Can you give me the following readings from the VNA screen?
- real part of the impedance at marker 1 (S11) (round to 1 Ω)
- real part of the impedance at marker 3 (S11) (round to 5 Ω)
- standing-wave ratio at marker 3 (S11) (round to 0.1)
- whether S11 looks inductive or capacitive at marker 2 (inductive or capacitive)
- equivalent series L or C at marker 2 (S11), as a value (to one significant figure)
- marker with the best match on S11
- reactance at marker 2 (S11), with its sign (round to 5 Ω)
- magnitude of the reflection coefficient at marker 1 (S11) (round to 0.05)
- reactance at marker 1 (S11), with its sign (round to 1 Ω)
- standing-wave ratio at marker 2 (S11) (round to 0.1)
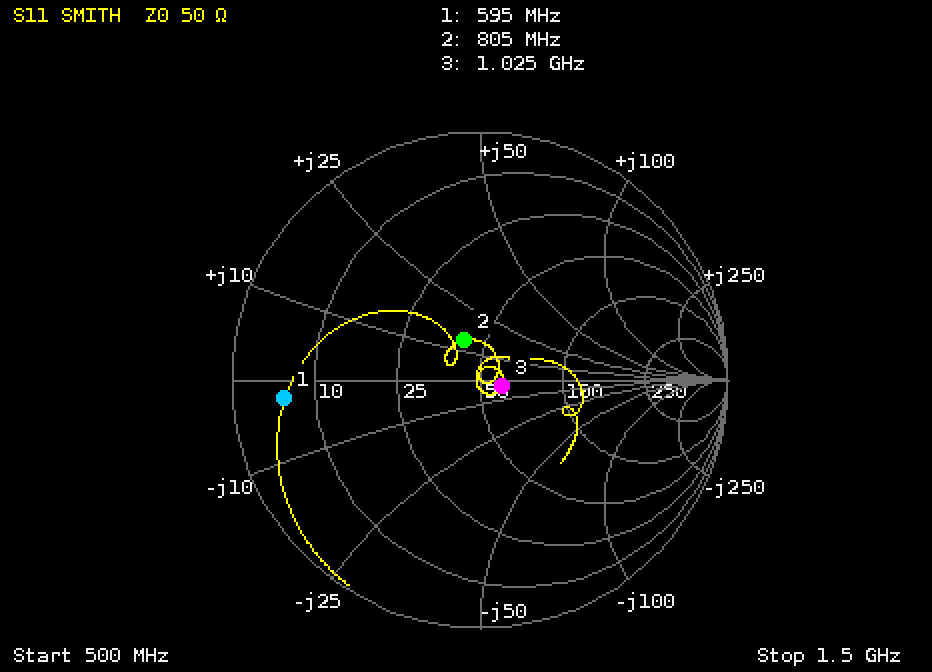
6 Ω
60 Ω
1.2
inductive
3 nH
marker 3
+15 Ω
0.80
-2 Ω
1.4
